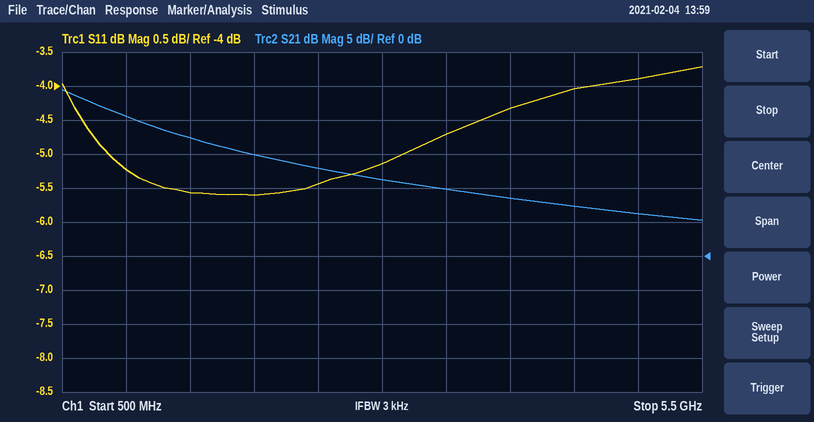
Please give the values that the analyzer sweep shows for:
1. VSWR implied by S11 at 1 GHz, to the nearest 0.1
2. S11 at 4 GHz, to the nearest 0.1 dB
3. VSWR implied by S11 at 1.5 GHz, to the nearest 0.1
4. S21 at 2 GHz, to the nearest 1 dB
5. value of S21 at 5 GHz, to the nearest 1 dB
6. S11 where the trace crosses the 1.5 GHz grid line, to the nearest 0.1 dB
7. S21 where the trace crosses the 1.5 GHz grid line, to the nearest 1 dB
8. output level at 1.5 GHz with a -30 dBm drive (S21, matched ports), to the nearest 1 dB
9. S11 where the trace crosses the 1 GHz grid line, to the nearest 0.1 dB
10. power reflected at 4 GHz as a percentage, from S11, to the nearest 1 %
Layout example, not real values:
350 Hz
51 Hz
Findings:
3.4
-4.3 dB
3.2
15 dB
6 dB
-5.6 dB
17 dB
-13 dBm
-5.2 dB
37 %
